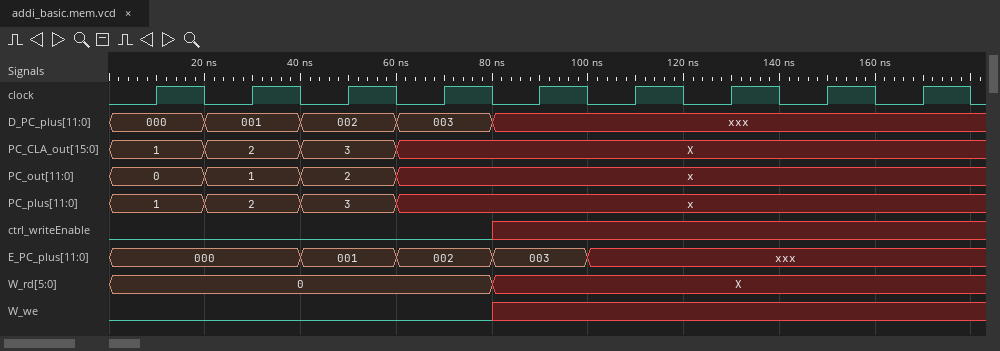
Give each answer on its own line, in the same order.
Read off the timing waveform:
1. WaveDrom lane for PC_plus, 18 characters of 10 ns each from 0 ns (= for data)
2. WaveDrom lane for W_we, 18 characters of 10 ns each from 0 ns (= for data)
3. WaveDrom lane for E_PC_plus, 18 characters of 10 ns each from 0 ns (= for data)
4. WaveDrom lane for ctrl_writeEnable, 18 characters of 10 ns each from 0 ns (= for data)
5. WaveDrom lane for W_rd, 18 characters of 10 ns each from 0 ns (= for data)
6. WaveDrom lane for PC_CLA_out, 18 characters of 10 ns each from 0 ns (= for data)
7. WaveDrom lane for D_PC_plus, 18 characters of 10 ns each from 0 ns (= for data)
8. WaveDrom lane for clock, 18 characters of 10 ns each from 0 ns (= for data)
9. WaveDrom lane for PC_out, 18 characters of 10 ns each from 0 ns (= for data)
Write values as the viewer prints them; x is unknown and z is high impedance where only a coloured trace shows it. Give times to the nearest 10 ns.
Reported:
{name: 'PC_plus', wave: '=.=.=.x...........', data: '1 2 3'}
{name: 'W_we', wave: '0.......x.........'}
{name: 'E_PC_plus', wave: '=...=.=.=.x.......', data: '000 001 002 003'}
{name: 'ctrl_writeEnable', wave: '0.......x.........'}
{name: 'W_rd', wave: '=.......=.........', data: '0 X'}
{name: 'PC_CLA_out', wave: '=.=.=.=...........', data: '1 2 3 X'}
{name: 'D_PC_plus', wave: '=.=.=.=.x.........', data: '000 001 002 003'}
{name: 'clock', wave: '010101010101010101'}
{name: 'PC_out', wave: '=.=.=.x...........', data: '0 1 2'}
